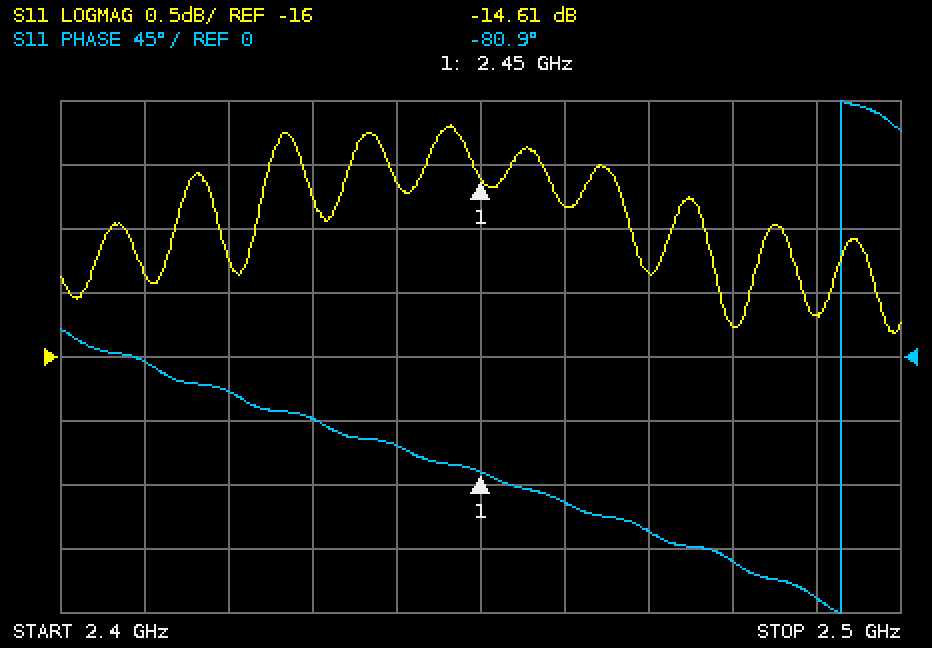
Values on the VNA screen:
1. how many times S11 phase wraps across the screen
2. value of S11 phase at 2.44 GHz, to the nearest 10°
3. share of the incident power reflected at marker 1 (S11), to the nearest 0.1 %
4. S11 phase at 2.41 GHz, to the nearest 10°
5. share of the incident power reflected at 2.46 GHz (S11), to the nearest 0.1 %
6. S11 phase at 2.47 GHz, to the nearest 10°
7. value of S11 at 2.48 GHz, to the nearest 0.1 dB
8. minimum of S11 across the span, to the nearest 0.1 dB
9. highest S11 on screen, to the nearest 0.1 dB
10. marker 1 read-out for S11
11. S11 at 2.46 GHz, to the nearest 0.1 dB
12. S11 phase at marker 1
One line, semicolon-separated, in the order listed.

1; -60°; 3.5 %; 0°; 3.3 %; -120°; -15.8 dB; -15.8 dB; -14.2 dB; -14.61 dB; -14.8 dB; -80.9°
